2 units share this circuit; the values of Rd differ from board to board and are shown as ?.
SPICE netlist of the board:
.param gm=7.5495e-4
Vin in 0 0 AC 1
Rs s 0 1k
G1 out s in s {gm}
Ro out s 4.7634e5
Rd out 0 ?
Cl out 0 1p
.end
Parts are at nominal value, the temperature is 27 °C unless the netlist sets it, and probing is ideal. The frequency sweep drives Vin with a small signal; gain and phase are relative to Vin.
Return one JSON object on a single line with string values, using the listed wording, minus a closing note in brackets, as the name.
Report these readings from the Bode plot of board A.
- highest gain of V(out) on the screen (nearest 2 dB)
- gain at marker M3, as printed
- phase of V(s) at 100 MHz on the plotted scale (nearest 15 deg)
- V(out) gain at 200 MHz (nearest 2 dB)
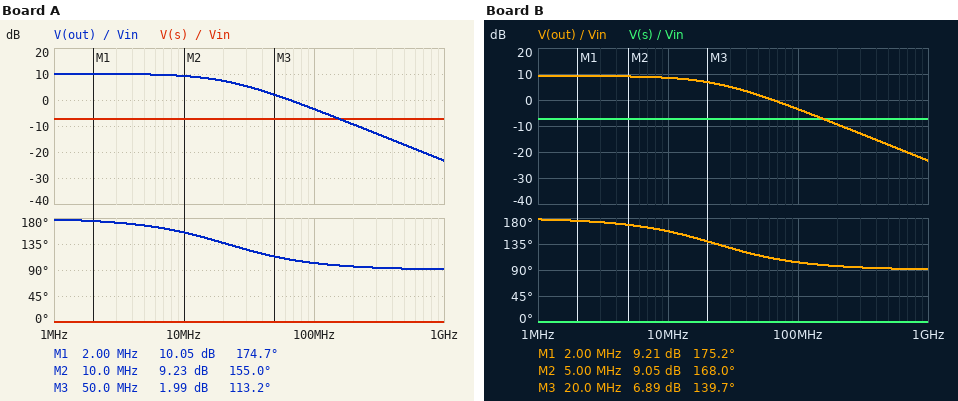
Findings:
{"highest gain of V(out) on the screen": "10 dB", "gain at marker M3, as printed": "1.99 dB", "phase of V(s) at 100 MHz on the plotted scale": "0 deg", "V(out) gain at 200 MHz": "-10 dB"}
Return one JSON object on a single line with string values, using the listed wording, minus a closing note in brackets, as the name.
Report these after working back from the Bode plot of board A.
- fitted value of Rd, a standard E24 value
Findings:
{"fitted value of Rd, a standard E24 value": "7.5 kΩ"}
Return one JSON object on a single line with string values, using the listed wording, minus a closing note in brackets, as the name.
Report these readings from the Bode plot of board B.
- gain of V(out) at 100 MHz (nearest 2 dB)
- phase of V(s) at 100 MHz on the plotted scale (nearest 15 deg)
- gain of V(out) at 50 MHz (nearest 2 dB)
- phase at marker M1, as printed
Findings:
{"gain of V(out) at 100 MHz": "-4 dB", "phase of V(s) at 100 MHz on the plotted scale": "0 deg", "gain of V(out) at 50 MHz": "2 dB", "phase at marker M1, as printed": "175.2 deg"}
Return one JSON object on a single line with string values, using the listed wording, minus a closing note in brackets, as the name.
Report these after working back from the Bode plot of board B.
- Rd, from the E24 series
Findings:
{"Rd, from the E24 series": "6.8 kΩ"}
